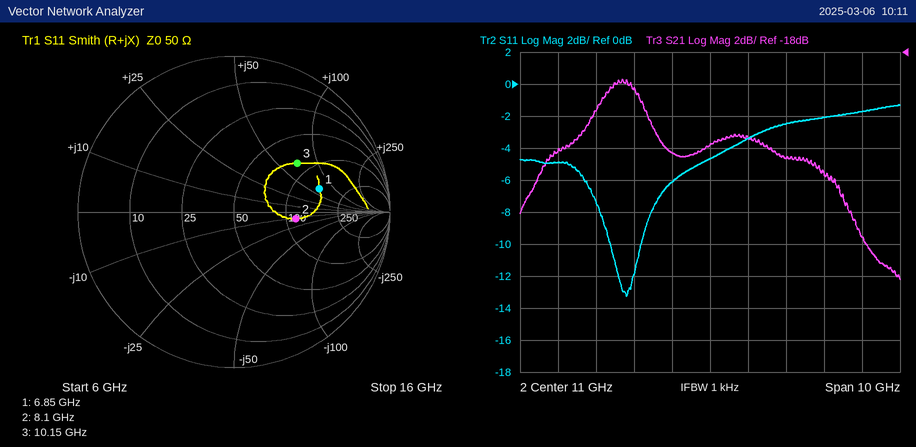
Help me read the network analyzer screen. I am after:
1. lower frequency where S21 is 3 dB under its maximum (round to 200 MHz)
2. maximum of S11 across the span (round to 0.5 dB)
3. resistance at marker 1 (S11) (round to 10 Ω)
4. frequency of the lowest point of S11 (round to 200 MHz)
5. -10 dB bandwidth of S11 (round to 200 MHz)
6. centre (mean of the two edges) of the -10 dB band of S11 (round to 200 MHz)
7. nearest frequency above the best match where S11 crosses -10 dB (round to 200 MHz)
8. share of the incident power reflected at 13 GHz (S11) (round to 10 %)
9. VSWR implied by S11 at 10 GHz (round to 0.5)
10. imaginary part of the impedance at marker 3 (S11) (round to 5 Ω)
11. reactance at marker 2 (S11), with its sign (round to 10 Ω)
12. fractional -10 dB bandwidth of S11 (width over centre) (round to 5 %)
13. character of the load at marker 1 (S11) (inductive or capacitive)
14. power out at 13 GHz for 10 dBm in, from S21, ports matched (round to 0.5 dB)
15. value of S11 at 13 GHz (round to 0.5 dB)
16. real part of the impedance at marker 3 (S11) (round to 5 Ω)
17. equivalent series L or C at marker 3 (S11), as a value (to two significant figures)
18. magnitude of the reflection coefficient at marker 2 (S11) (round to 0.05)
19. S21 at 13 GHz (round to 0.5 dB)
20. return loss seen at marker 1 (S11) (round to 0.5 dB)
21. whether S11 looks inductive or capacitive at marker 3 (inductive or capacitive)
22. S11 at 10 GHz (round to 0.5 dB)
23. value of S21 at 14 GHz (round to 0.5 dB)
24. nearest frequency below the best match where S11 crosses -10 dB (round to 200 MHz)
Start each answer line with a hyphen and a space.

- 7.8 GHz
- -1.5 dB
- 150 Ω
- 8.8 GHz
- 800 MHz
- 8.8 GHz
- 9.2 GHz
- 60 %
- 3.0
- +70 Ω
- -10 Ω
- 10 %
- inductive
- -14.5 dBm
- -2.5 dB
- 80 Ω
- 1.1 nH
- 0.40
- -24.5 dB
- 5.0 dB
- inductive
- -6.0 dB
- -25.5 dB
- 8.4 GHz
